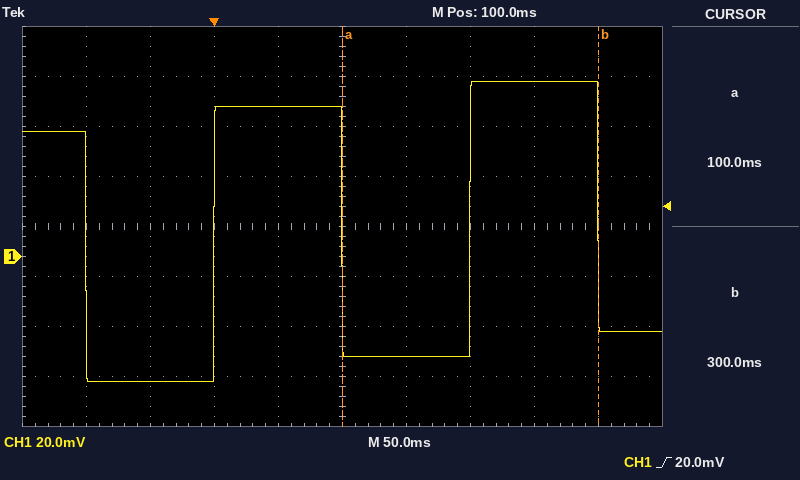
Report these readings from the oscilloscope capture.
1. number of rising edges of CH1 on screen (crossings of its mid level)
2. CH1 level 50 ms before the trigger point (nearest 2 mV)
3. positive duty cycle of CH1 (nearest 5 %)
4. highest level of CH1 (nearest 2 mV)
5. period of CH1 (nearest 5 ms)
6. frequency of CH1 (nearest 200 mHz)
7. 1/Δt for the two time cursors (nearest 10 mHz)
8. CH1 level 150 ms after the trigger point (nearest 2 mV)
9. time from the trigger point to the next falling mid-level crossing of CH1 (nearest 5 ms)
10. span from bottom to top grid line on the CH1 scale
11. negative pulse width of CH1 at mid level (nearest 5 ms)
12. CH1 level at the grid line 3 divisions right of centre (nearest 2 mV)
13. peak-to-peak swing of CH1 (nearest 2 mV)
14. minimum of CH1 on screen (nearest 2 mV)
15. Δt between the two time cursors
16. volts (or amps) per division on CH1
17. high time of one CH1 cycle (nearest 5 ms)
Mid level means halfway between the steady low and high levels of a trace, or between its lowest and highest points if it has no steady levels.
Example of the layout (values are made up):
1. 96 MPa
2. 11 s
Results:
1. 2
2. -50 mV
3. 50 %
4. 70 mV
5. 200 ms
6. 5.0 Hz
7. 5.00 Hz
8. -40 mV
9. 100 ms
10. 160 mV
11. 100 ms
12. 70 mV
13. 120 mV
14. -50 mV
15. 200 ms
16. 20 mV
17. 100 ms
